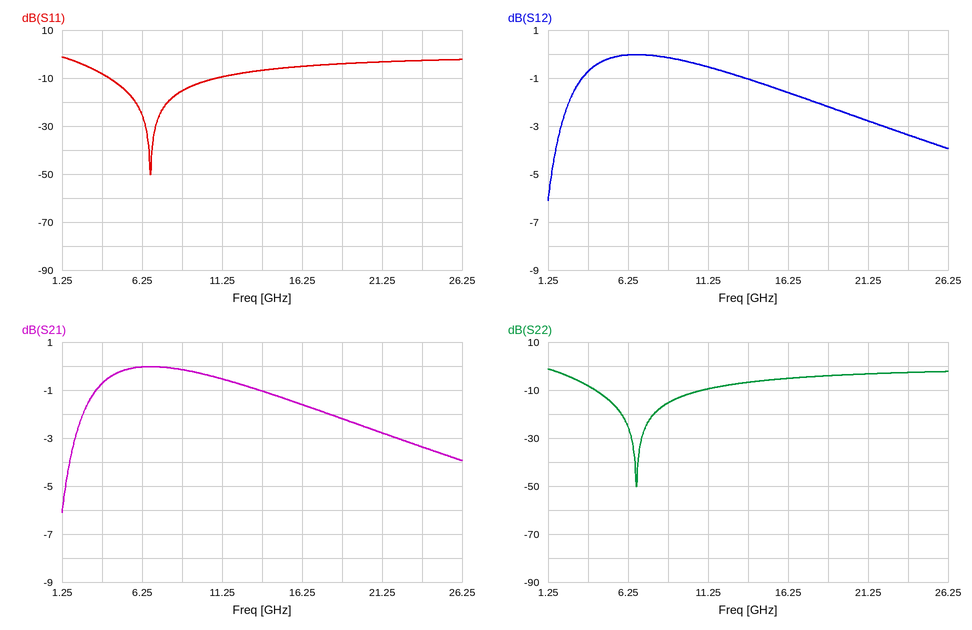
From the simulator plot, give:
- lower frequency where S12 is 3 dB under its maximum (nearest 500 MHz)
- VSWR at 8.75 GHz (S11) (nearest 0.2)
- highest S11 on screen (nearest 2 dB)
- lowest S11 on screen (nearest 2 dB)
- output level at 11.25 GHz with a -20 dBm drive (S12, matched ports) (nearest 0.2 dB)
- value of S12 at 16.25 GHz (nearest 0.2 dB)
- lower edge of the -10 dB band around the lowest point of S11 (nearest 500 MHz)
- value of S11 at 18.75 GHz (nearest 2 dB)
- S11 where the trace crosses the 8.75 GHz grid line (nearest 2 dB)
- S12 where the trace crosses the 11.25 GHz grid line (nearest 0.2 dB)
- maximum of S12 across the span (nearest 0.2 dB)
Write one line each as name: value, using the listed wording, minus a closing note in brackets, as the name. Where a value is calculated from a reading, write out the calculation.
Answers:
lower frequency where S12 is 3 dB under its maximum: 2.0 GHz
VSWR at 8.75 GHz (S11): |Γ| = 10^(-16/20) = 0.1585; VSWR = (1 + 0.1585)/(1 − 0.1585) ≈ 1.4
highest S11 on screen: -2 dB
lowest S11 on screen: -50 dB
output level at 11.25 GHz with a -20 dBm drive (S12, matched ports): -20 dBm + (-0.6 dB) = -20.6 dBm
value of S12 at 16.25 GHz: -1.6 dB
lower edge of the -10 dB band around the lowest point of S11: 4.0 GHz
value of S11 at 18.75 GHz: -4 dB
S11 where the trace crosses the 8.75 GHz grid line: -16 dB
S12 where the trace crosses the 11.25 GHz grid line: -0.6 dB
maximum of S12 across the span: 0.0 dB
